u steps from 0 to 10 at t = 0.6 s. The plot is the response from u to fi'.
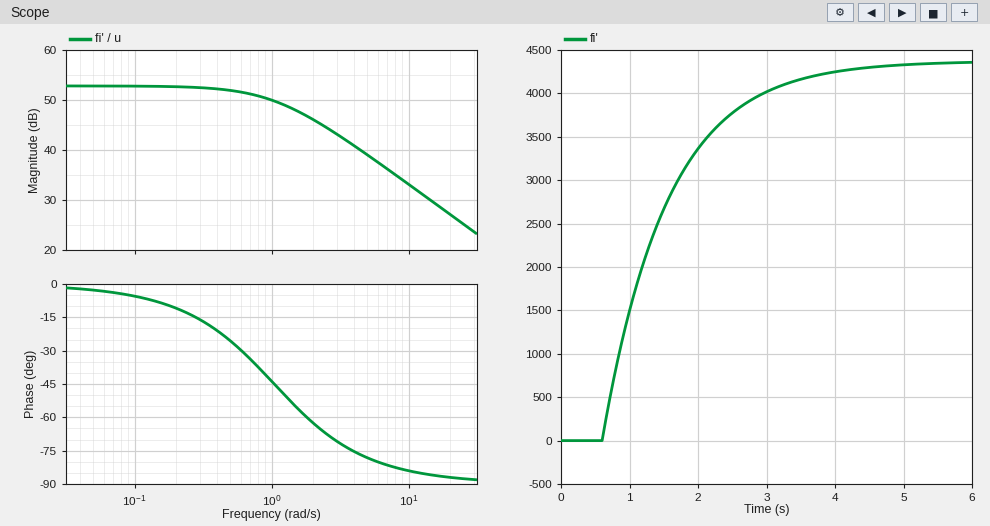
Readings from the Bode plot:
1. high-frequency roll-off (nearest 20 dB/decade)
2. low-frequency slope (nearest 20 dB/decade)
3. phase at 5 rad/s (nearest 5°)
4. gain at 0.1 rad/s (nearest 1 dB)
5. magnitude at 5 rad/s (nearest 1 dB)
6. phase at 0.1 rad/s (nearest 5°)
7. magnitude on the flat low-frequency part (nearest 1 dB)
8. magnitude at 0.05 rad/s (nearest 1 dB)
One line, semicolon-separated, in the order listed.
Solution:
-20 dB/decade; 0 dB/decade; -80°; 53 dB; 39 dB; -5°; 53 dB; 53 dB
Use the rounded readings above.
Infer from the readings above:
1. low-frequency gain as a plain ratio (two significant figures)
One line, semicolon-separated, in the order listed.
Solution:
450
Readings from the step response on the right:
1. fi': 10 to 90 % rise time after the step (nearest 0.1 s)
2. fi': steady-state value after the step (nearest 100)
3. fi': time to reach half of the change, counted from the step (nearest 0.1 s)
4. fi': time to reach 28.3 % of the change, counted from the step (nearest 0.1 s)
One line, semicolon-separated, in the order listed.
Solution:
2.1 s; 4400; 0.7 s; 0.3 s
